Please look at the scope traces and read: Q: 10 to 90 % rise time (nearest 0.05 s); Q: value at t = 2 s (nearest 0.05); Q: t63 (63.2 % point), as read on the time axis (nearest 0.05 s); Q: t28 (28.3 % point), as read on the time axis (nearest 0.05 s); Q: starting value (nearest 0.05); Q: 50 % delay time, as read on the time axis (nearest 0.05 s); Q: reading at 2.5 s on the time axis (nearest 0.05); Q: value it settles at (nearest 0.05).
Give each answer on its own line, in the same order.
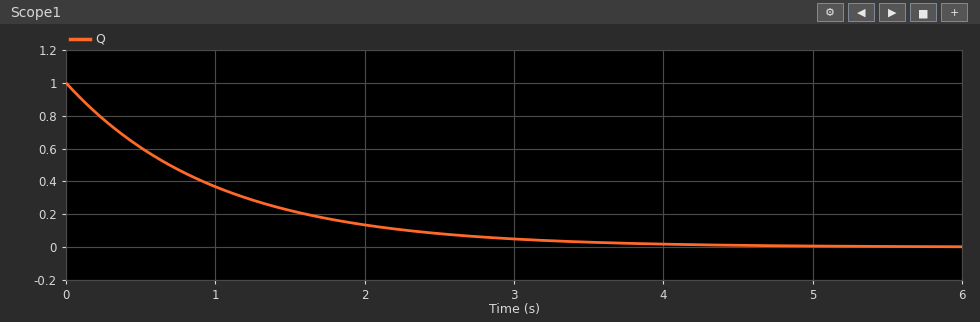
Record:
2.20 s
0.15
1.00 s
0.35 s
1.00
0.70 s
0.10
0.00
